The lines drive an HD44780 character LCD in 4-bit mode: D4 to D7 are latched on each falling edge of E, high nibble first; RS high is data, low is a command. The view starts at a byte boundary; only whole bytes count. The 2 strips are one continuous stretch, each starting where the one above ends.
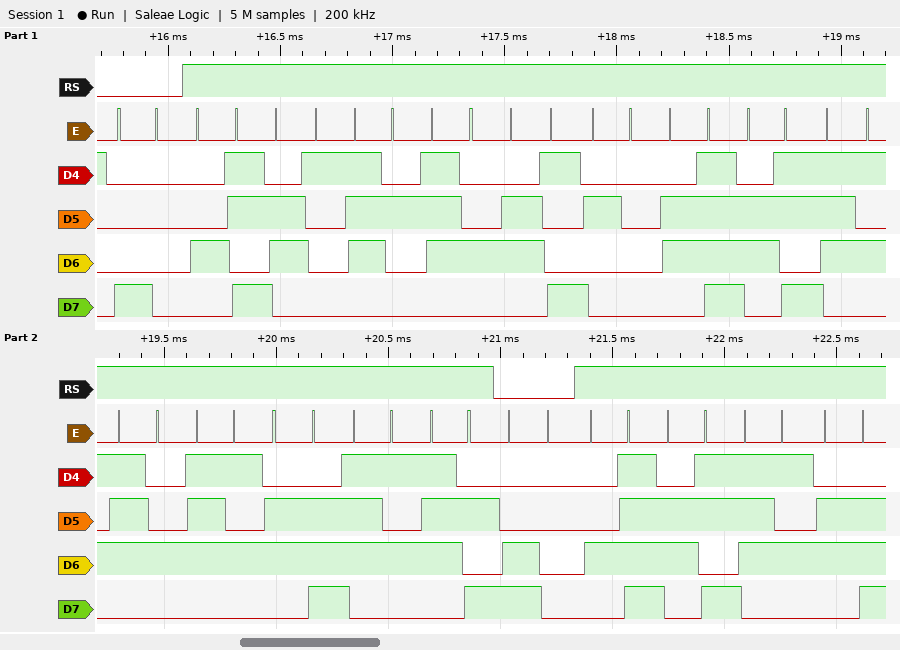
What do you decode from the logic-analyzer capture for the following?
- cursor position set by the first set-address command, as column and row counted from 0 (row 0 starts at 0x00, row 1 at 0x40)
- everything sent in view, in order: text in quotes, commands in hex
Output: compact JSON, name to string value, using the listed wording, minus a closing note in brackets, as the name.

{"cursor position set by the first set-address command, as column and row counted from 0": "column 0, row 0", "everything sent in view, in order: text in quotes, commands in hex": "0x80 \"Karti okutunuz\" 0xC0 \"Okun\""}
